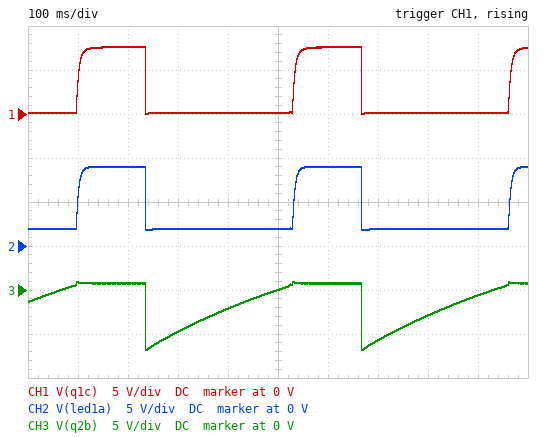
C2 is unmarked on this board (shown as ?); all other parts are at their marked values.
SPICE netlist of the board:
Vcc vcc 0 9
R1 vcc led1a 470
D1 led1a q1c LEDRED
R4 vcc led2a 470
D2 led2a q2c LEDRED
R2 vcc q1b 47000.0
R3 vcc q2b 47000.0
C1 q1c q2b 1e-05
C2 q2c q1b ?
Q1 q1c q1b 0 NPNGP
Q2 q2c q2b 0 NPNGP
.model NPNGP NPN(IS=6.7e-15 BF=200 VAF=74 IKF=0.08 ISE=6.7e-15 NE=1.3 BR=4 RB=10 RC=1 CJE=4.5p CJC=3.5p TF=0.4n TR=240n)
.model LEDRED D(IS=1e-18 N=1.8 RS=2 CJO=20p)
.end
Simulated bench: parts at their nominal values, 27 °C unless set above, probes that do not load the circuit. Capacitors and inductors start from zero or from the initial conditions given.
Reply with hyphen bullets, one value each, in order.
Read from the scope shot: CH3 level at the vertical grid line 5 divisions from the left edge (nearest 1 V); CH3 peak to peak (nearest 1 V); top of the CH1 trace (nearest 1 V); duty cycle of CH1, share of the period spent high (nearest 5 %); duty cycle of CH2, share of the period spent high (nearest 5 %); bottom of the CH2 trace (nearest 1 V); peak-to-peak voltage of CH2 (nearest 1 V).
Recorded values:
- 0 V
- 8 V
- 8 V
- 30 %
- 30 %
- 2 V
- 7 V
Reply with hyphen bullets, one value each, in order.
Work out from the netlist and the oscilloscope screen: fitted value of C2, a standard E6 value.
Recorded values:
- 4.7 µF
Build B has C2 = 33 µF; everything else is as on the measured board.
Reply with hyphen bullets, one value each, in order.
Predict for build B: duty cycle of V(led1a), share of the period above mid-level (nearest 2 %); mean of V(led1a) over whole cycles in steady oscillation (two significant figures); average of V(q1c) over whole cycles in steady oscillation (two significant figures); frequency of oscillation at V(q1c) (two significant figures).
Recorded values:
- 76 %
- 7.3 V
- 5.9 V
- 790 mHz
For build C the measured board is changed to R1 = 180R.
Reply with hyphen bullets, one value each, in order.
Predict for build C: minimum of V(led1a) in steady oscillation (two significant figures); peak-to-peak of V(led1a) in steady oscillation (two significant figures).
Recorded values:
- 1.9 V
- 7.1 V
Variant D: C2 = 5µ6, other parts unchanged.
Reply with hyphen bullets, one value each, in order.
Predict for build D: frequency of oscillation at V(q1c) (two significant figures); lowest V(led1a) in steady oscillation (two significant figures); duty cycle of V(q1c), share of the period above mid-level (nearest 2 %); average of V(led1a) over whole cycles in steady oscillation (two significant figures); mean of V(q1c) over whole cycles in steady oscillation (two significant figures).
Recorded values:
- 2.2 Hz
- 1.8 V
- 36 %
- 4.4 V
- 2.7 V
